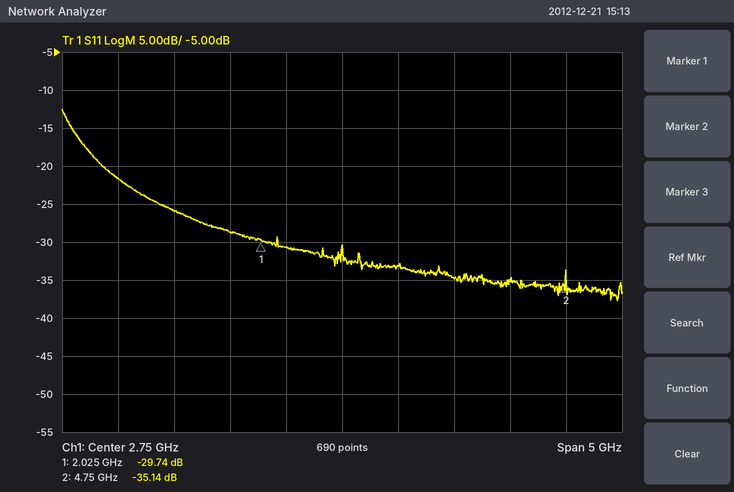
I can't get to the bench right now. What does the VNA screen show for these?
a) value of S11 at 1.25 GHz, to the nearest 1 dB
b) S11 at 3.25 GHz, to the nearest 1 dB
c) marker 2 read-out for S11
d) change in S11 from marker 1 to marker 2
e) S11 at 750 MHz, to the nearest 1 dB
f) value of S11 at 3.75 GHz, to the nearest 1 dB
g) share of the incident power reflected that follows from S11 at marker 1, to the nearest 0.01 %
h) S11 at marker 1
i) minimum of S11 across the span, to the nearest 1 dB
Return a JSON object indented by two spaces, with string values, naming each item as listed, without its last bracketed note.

{
  "value of S11 at 1.25 GHz, to the nearest 1 dB": "-26 dB",
  "S11 at 3.25 GHz, to the nearest 1 dB": "-33 dB",
  "marker 2 read-out for S11": "-35.14 dB",
  "change in S11 from marker 1 to marker 2": "-5.40 dB",
  "S11 at 750 MHz, to the nearest 1 dB": "-22 dB",
  "value of S11 at 3.75 GHz, to the nearest 1 dB": "-35 dB",
  "share of the incident power reflected that follows from S11 at marker 1, to the nearest 0.01 %": "0.11 %",
  "S11 at marker 1": "-29.74 dB",
  "minimum of S11 across the span, to the nearest 1 dB": "-38 dB"
}
